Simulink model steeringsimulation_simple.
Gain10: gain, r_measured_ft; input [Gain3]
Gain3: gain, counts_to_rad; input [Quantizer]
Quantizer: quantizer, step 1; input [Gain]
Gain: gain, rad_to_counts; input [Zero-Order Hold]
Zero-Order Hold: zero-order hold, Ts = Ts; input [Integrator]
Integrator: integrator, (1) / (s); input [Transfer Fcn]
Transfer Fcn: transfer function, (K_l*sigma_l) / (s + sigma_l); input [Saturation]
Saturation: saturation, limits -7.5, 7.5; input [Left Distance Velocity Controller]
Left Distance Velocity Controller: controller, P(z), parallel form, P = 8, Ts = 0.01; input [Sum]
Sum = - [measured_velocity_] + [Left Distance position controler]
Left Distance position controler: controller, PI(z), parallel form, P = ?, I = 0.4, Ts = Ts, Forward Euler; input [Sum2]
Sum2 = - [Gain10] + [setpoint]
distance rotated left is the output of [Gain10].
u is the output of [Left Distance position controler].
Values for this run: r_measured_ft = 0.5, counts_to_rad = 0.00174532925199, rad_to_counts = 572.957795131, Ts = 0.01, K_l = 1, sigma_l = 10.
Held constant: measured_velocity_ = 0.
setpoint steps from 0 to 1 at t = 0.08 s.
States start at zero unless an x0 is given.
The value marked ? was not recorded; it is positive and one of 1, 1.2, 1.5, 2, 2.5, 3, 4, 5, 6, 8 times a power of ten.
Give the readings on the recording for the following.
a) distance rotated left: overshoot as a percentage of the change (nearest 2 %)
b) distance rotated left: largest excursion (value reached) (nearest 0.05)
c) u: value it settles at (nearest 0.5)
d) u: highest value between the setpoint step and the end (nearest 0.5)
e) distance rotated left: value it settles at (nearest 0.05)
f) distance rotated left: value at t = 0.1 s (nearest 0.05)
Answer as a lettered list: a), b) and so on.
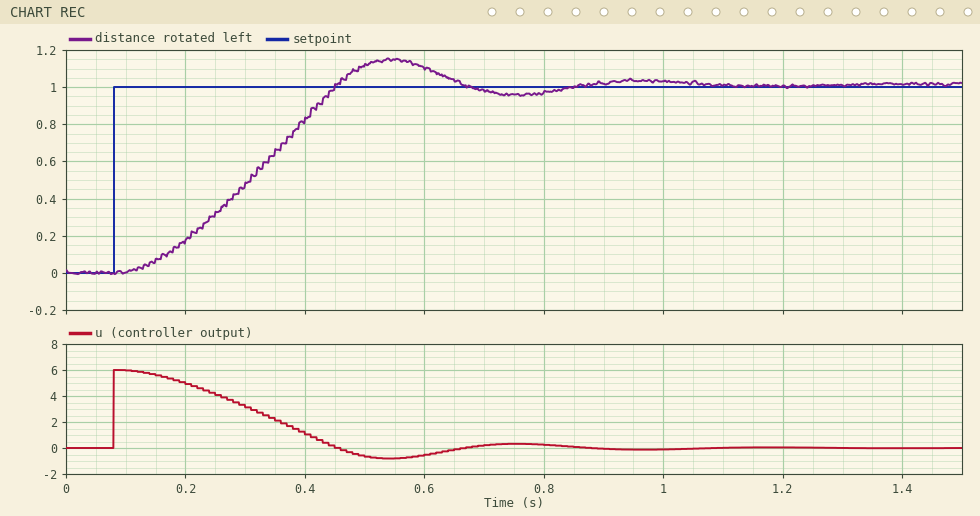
a) 14 %
b) 1.15
c) 0.0
d) 6.0
e) 1.00
f) 0.00
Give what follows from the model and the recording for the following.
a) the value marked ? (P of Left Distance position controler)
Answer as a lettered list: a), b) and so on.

a) 6
